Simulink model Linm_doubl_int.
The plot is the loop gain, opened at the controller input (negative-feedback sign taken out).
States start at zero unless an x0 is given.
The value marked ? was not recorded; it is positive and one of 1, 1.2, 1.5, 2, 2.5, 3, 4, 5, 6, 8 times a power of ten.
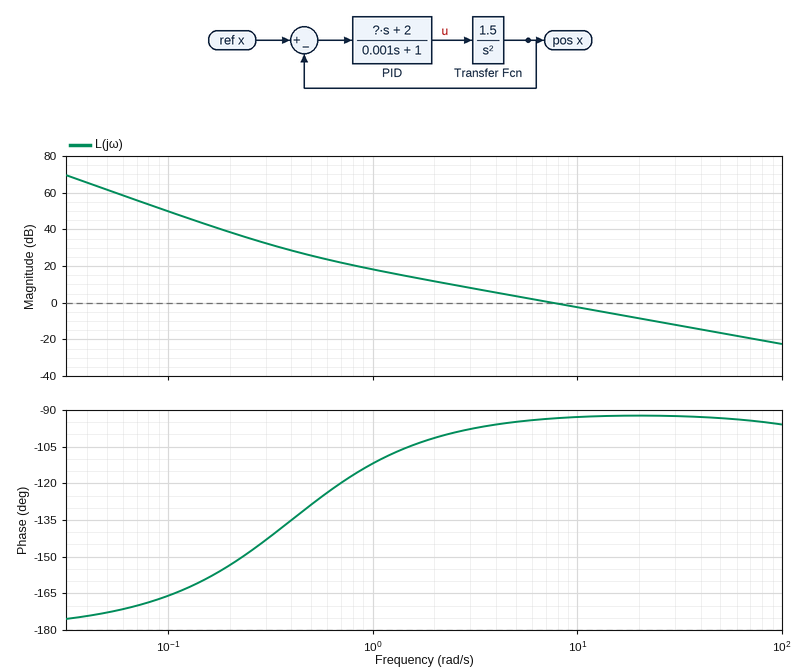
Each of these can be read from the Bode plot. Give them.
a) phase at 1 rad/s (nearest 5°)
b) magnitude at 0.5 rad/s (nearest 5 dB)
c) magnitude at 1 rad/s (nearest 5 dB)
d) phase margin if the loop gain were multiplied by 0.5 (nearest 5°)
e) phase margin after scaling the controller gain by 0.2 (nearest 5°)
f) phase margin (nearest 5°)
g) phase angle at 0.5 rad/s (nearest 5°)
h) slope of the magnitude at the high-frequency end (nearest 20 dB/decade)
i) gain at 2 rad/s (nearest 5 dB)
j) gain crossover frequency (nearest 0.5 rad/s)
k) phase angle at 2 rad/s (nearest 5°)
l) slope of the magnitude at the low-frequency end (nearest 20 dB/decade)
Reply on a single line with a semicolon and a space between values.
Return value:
-110°; 25 dB; 20 dB; 85°; 75°; 85°; -130°; -20 dB/decade; 10 dB; 7.5 rad/s; -100°; -40 dB/decade
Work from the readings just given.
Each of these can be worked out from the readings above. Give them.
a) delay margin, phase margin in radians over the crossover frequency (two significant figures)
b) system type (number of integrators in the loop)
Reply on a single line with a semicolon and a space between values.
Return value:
0.20 s; 2
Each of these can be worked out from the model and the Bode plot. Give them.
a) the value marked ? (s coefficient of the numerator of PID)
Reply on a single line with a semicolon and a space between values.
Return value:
5
